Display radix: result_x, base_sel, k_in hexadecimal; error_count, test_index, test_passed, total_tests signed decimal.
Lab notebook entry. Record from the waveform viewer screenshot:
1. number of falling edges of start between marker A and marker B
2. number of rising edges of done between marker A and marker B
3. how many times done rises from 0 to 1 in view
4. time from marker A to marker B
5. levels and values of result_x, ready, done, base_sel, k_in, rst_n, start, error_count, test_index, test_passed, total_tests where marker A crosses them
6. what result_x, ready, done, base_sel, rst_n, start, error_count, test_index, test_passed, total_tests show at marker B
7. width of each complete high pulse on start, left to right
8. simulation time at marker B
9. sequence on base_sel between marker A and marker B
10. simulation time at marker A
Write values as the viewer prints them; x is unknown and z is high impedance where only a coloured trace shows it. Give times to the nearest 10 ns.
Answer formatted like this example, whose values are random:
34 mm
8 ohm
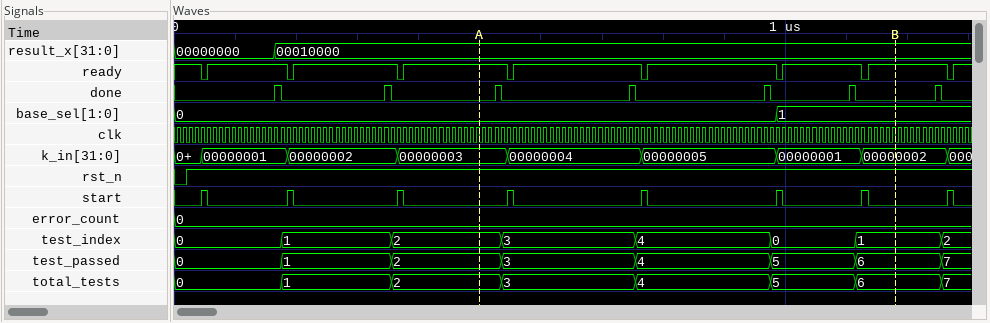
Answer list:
4
4
7
680 ns
result_x=00010000, ready=1, done=0, base_sel=0, k_in=00000003, rst_n=1, start=0, error_count=0, test_index=2, test_passed=2, total_tests=2
result_x=00010000, ready=1, done=0, base_sel=1, rst_n=1, start=0, error_count=0, test_index=1, test_passed=6, total_tests=6
10 ns, 10 ns, 10 ns, 10 ns, 10 ns, 10 ns, 10 ns, 10 ns
1180 ns
0, 1
500 ns
